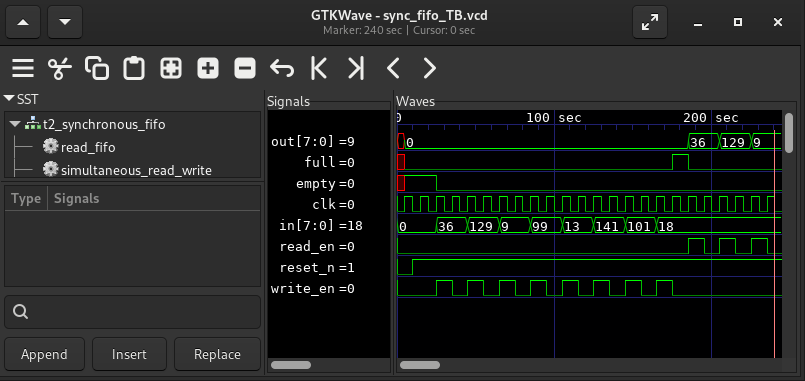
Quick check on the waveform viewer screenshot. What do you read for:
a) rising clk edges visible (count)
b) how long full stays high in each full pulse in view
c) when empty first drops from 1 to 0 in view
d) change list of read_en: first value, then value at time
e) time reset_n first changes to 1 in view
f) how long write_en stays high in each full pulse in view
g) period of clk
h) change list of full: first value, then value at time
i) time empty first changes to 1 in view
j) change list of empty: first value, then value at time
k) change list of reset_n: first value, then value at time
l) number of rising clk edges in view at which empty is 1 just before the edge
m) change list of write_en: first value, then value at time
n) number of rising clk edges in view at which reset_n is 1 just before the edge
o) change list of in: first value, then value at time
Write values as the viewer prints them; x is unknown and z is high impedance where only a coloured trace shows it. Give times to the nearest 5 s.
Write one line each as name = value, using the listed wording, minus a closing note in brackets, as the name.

rising clk edges visible = 24
how long full stays high in each full pulse in view = 10 s
when empty first drops from 1 to 0 in view = 25 s
change list of read_en: first value, then value at time = 0, 1 at 185 s, 0 at 195 s, 1 at 205 s, 0 at 215 s, 1 at 225 s, 0 at 235 s
time reset_n first changes to 1 in view = 10 s
how long write_en stays high in each full pulse in view = 10 s, 10 s, 10 s, 10 s, 10 s, 10 s, 10 s, 10 s
period of clk = 10 s
change list of full: first value, then value at time = x, 0 at 5 s, 1 at 175 s, 0 at 185 s
time empty first changes to 1 in view = 5 s
change list of empty: first value, then value at time = x, 1 at 5 s, 0 at 25 s
change list of reset_n: first value, then value at time = 0, 1 at 10 s
number of rising clk edges in view at which empty is 1 just before the edge = 2
change list of write_en: first value, then value at time = 0, 1 at 25 s, 0 at 35 s, 1 at 45 s, 0 at 55 s, 1 at 65 s, 0 at 75 s, 1 at 85 s, 0 at 95 s, 1 at 105 s, 0 at 115 s, 1 at 125 s, 0 at 135 s, 1 at 145 s, 0 at 155 s, 1 at 165 s, 0 at 175 s
number of rising clk edges in view at which reset_n is 1 just before the edge = 23
change list of in: first value, then value at time = 0, 36 at 25 s, 129 at 45 s, 9 at 65 s, 99 at 85 s, 13 at 105 s, 141 at 125 s, 101 at 145 s, 18 at 165 s
